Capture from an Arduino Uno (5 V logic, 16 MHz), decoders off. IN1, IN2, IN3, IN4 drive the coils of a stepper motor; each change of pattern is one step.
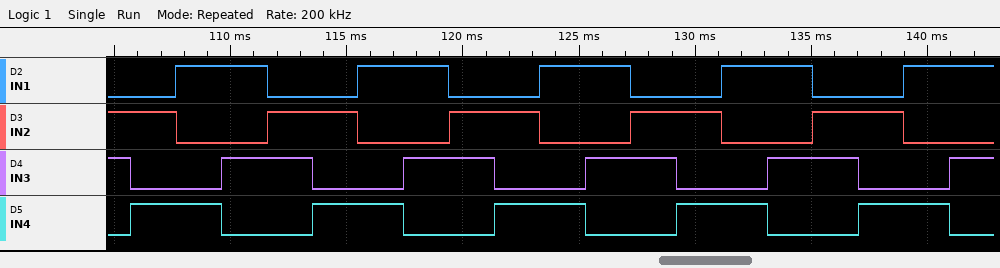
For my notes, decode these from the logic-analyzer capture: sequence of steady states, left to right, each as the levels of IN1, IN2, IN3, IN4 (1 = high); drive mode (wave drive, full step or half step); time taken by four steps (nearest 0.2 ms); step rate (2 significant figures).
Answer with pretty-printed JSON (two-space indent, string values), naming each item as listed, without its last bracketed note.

{
  "sequence of steady states, left to right, each as the levels of IN1, IN2, IN3, IN4": "0110 0101 1001 1010 0110 0101 1001 1010 0110 0101 1001 1010 0110 0101 1001 1010 0110 0101 1001 1010",
  "drive mode": "full step",
  "time taken by four steps": "7.8 ms",
  "step rate": "510 steps/s"
}
